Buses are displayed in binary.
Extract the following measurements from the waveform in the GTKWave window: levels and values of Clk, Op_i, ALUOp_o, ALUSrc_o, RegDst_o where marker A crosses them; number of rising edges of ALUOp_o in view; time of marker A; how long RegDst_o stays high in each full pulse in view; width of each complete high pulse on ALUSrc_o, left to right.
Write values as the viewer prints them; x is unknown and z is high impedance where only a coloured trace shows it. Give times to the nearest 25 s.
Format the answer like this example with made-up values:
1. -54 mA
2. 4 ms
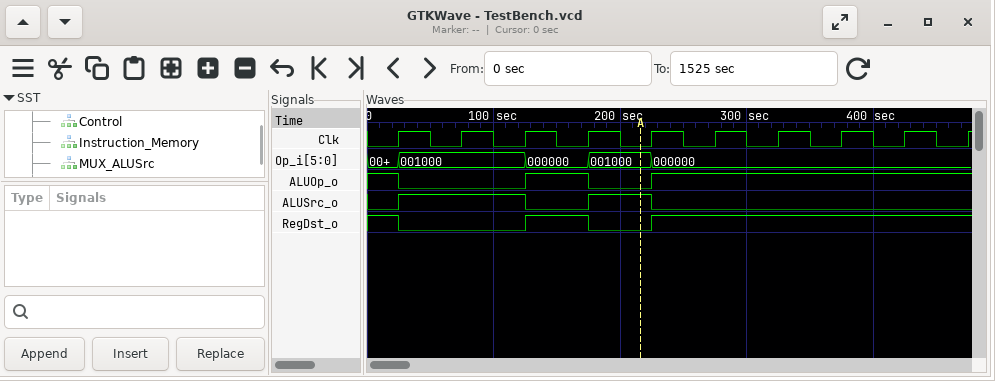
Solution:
1. Clk=0, Op_i=001000, ALUOp_o=0, ALUSrc_o=1, RegDst_o=0
2. 2
3. 225 s
4. 50 s
5. 100 s, 50 s
